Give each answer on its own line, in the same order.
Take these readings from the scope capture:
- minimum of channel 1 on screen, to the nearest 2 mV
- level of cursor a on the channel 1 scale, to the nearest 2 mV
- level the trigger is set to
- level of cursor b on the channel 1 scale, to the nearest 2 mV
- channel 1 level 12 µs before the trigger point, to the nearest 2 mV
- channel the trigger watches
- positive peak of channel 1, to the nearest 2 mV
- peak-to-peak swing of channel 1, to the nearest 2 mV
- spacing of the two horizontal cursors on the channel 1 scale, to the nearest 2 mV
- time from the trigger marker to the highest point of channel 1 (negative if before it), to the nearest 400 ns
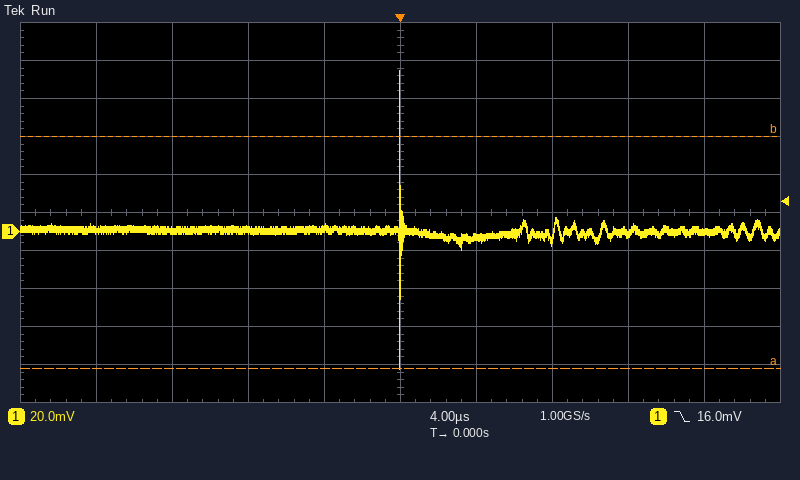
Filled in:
-72 mV
-72 mV
16.0 mV
50 mV
0 mV
channel 1
84 mV
156 mV
122 mV
0.0 µs
